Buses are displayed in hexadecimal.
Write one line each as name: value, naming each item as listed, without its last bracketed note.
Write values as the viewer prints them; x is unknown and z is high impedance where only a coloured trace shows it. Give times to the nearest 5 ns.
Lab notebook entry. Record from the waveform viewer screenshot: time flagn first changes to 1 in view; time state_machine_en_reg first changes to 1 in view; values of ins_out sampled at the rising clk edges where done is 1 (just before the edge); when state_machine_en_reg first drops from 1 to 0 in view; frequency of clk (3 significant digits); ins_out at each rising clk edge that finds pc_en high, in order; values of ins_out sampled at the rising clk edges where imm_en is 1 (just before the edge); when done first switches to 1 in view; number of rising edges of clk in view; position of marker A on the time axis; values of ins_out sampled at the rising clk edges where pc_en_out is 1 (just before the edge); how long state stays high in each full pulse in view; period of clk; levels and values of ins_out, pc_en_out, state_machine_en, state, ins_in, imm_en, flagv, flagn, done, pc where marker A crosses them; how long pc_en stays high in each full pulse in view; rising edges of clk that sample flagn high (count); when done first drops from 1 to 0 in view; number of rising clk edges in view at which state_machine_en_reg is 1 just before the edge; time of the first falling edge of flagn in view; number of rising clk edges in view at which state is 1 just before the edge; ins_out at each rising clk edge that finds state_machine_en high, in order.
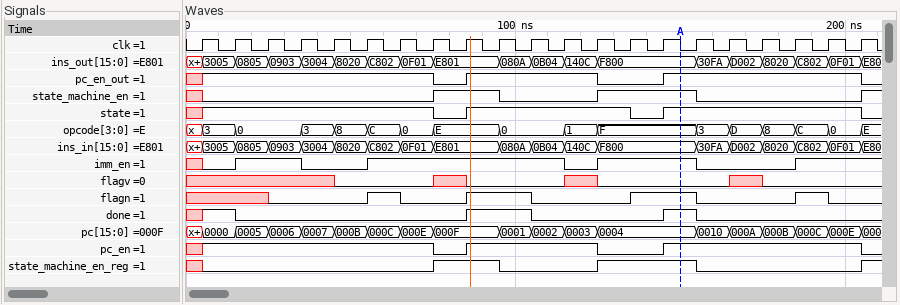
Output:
time flagn first changes to 1 in view: 55 ns
time state_machine_en_reg first changes to 1 in view: 75 ns
values of ins_out sampled at the rising clk edges where done is 1: 3005, E801, 080A, F800
when state_machine_en_reg first drops from 1 to 0 in view: 95 ns
frequency of clk: 100 MHz
ins_out at each rising clk edge that finds pc_en high, in order: 3005, 0805, 0903, 3004, 8020, C802, 0F01, E801, 080A, 0B04, 140C, F800, 30FA, D002, 8020, C802, 0F01
values of ins_out sampled at the rising clk edges where imm_en is 1: 0805, 0903, C802, 0F01, E801, E801, 080A, 0B04, F800, F800, F800, C802, 0F01
when done first switches to 1 in view: 5 ns
number of rising edges of clk in view: 21
position of marker A on the time axis: 150 ns
values of ins_out sampled at the rising clk edges where pc_en_out is 1: 3005, 0805, 0903, 3004, 8020, C802, 0F01, E801, 080A, 0B04, 140C, F800, 30FA, D002, 8020, C802, 0F01
how long state stays high in each full pulse in view: 50 ns, 60 ns
period of clk: 10 ns
levels and values of ins_out, pc_en_out, state_machine_en, state, ins_in, imm_en, flagv, flagn, done, pc where marker A crosses them: ins_out=F800, pc_en_out=1, state_machine_en=1, state=1, ins_in=F800, imm_en=1, flagv=0, flagn=1, done=1, pc=0004
how long pc_en stays high in each full pulse in view: 40 ns, 60 ns
rising edges of clk that sample flagn high: 6
when done first drops from 1 to 0 in view: 15 ns
number of rising clk edges in view at which state_machine_en_reg is 1 just before the edge: 5
time of the first falling edge of flagn in view: 65 ns
number of rising clk edges in view at which state is 1 just before the edge: 18
ins_out at each rising clk edge that finds state_machine_en high, in order: E801, E801, F800, F800, F800
